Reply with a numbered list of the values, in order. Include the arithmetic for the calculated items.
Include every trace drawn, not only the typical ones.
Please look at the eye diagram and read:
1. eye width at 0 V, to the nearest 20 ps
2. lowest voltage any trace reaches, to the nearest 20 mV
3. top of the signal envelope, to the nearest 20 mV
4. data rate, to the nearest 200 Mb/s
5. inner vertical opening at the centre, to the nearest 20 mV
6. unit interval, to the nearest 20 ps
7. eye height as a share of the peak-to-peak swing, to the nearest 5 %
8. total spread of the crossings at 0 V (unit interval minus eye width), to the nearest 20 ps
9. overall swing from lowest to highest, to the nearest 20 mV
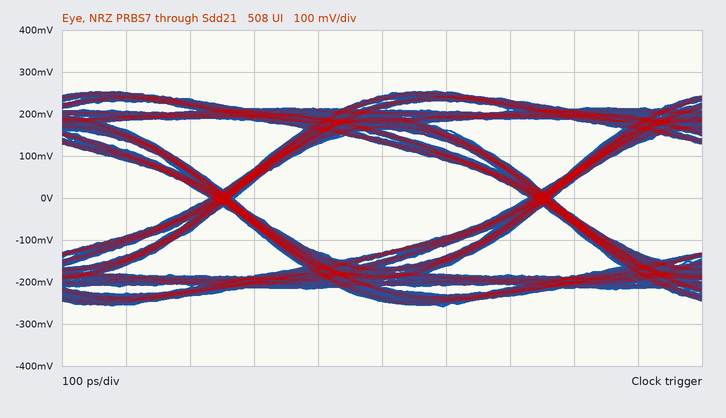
1. 460 ps
2. -260 mV
3. 260 mV
4. 2.0 Gb/s
5. 260 mV
6. 500 ps
7. 260 mV / 520 mV ≈ 50 %
8. 40 ps
9. 520 mV
